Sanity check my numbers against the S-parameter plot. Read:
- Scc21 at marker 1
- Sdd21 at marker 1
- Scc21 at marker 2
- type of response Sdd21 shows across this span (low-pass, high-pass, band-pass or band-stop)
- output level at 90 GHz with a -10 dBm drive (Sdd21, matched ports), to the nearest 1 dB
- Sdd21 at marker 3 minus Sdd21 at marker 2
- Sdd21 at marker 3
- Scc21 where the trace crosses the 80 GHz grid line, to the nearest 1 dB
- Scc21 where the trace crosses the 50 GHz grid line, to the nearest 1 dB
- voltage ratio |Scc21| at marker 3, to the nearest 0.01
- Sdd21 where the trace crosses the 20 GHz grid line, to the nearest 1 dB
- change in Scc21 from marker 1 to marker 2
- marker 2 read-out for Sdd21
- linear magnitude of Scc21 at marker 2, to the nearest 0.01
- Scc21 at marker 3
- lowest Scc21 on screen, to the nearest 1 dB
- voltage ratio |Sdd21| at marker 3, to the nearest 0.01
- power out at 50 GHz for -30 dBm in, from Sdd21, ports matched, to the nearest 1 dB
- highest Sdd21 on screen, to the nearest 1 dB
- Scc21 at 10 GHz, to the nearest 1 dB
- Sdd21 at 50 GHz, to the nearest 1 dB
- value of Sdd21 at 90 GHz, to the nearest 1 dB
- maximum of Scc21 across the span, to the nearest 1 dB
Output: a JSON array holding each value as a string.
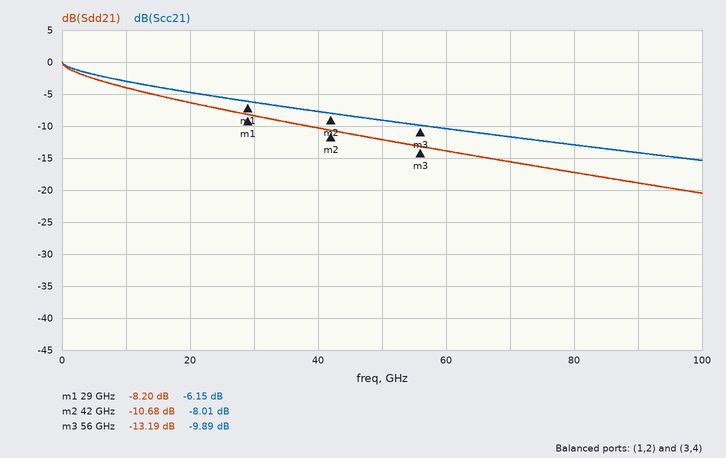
["-6.15 dB", "-8.20 dB", "-8.01 dB", "low-pass", "-29 dBm", "-2.51 dB", "-13.19 dB", "-13 dB", "-9 dB", "0.32", "-6 dB", "-1.86 dB", "-10.68 dB", "0.40", "-9.89 dB", "-15 dB", "0.22", "-42 dBm", "0 dB", "-3 dB", "-12 dB", "-19 dB", "0 dB"]
